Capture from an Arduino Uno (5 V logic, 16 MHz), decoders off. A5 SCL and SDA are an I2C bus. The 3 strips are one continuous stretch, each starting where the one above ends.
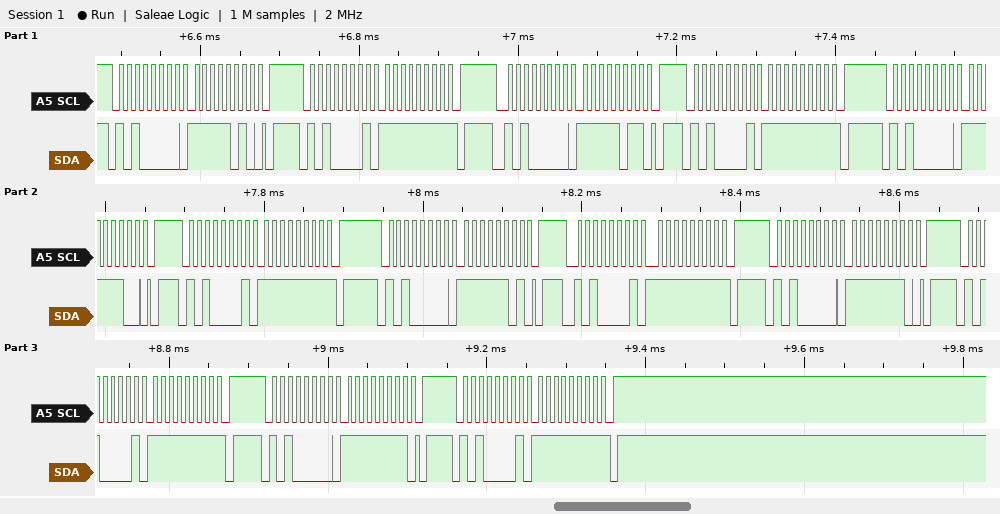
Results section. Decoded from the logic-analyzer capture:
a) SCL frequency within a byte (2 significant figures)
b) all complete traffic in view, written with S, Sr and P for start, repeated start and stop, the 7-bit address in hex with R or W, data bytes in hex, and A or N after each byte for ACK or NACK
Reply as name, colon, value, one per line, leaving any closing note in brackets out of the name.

SCL frequency within a byte: 100 kHz
all complete traffic in view, written with S, Sr and P for start, repeated start and stop, the 7-bit address in hex with R or W, data bytes in hex, and A or N after each byte for ACK or NACK: S 50W A FA A P S 50R A FF N P S 50W A FB A P S 50R A FF N P S 50W A FC A P S 50R A FF N P S 50W A FD A P S 50R A FF N P S 50W A FE A P S 50R A FF N P S 50W A FF A P S 50R A FF N P
